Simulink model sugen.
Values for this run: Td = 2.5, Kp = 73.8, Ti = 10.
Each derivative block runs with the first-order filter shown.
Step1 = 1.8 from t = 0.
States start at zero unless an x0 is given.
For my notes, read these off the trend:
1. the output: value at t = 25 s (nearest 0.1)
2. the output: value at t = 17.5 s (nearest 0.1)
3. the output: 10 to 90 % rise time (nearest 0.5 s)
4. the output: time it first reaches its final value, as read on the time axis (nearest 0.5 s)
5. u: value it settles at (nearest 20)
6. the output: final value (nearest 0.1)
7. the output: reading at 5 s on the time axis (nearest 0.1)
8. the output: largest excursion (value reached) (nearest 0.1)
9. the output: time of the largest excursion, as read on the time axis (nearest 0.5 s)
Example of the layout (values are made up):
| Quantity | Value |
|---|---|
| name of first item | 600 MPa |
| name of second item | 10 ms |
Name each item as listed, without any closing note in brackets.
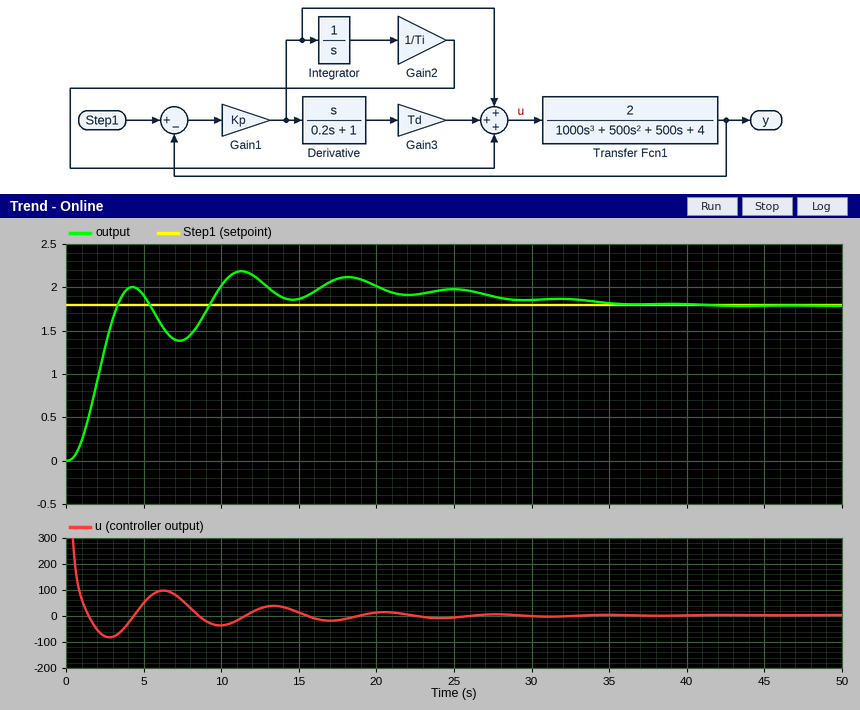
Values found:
| Quantity | Value |
|---|---|
| the output: value at t = 25 s | 2.0 |
| the output: value at t = 17.5 s | 2.1 |
| the output: 10 to 90 % rise time | 2.0 s |
| the output: time it first reaches its final value, as read on the time axis | 3.5 s |
| u: value it settles at | 0 |
| the output: final value | 1.8 |
| the output: reading at 5 s on the time axis | 1.9 |
| the output: largest excursion (value reached) | 2.2 |
| the output: time of the largest excursion, as read on the time axis | 11.5 s |
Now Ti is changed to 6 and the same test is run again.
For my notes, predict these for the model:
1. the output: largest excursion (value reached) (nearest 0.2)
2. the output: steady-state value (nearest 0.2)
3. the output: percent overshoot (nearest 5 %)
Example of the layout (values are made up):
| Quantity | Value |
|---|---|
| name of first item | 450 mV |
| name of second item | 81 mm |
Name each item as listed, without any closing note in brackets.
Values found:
| Quantity | Value |
|---|---|
| the output: largest excursion (value reached) | 2.4 |
| the output: steady-state value | 1.8 |
| the output: percent overshoot | 30 % |
